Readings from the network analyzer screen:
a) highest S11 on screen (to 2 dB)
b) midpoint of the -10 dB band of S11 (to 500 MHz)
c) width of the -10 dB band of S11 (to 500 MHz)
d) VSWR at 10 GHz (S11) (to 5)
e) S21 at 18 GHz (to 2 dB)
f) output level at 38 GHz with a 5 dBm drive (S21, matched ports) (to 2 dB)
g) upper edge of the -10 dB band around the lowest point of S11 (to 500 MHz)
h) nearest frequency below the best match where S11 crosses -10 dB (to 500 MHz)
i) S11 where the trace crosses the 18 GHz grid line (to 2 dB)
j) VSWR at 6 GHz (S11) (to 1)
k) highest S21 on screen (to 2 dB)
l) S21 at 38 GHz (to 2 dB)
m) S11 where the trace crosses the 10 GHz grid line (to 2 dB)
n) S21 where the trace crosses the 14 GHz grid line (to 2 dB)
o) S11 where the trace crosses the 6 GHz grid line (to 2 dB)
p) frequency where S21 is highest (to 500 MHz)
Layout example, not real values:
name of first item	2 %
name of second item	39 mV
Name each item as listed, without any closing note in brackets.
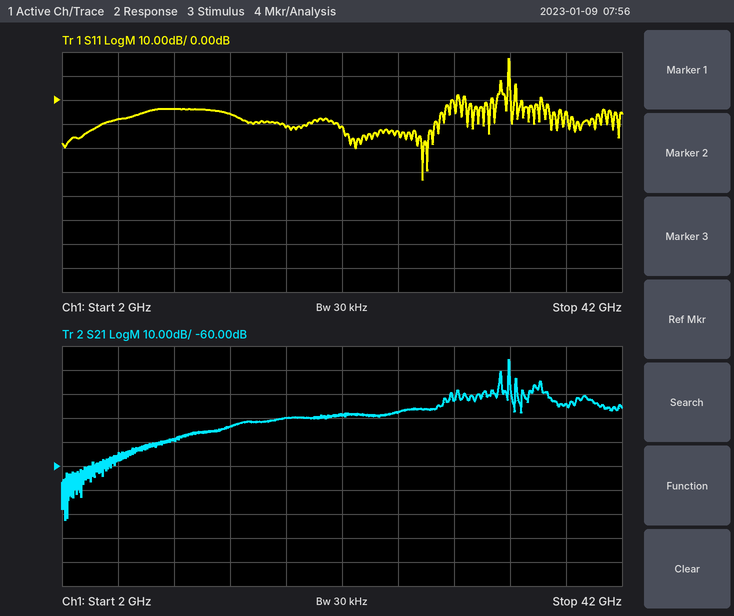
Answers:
highest S11 on screen	18 dB
midpoint of the -10 dB band of S11	25.0 GHz
width of the -10 dB band of S11	7.0 GHz
VSWR at 10 GHz (S11)	5
S21 at 18 GHz	-40 dB
output level at 38 GHz with a 5 dBm drive (S21, matched ports)	-30 dBm
upper edge of the -10 dB band around the lowest point of S11	28.5 GHz
nearest frequency below the best match where S11 crosses -10 dB	21.5 GHz
S11 where the trace crosses the 18 GHz grid line	-12 dB
VSWR at 6 GHz (S11)	2
highest S21 on screen	-16 dB
S21 at 38 GHz	-34 dB
S11 where the trace crosses the 10 GHz grid line	-4 dB
S21 where the trace crosses the 14 GHz grid line	-44 dB
S11 where the trace crosses the 6 GHz grid line	-8 dB
frequency where S21 is highest	34.0 GHz
